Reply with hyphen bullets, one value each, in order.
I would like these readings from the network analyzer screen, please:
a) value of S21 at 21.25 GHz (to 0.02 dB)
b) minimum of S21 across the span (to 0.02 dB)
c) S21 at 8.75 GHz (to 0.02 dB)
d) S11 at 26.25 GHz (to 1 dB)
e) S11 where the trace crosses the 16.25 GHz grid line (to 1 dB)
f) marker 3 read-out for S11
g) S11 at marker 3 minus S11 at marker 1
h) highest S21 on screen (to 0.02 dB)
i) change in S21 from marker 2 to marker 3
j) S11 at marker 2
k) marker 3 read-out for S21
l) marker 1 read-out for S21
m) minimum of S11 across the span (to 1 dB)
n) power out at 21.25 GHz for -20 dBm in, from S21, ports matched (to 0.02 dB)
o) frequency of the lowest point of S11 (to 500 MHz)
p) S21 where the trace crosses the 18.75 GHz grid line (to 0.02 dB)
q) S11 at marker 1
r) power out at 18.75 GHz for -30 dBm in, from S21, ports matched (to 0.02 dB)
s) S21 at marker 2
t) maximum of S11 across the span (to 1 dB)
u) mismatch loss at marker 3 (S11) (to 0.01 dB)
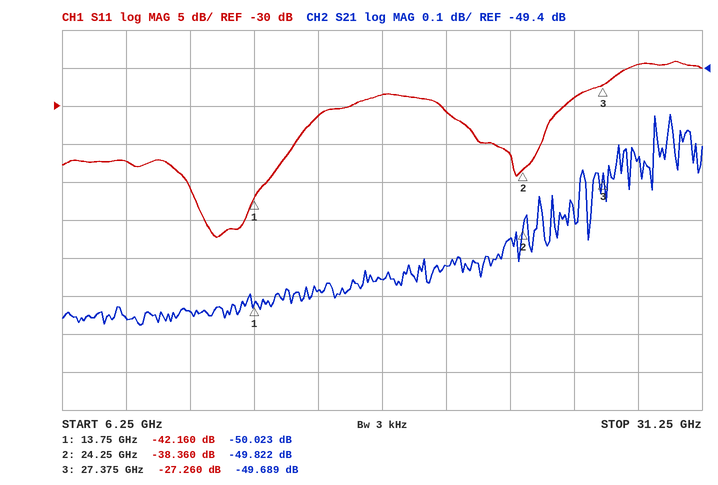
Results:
- -49.92 dB
- -50.08 dB
- -50.06 dB
- -29 dB
- -31 dB
- -27.260 dB
- 14.900 dB
- -49.52 dB
- 0.133 dB
- -38.360 dB
- -49.689 dB
- -50.023 dB
- -47 dB
- -69.92 dBm
- 12.5 GHz
- -49.96 dB
- -42.160 dB
- -79.96 dBm
- -49.822 dB
- -24 dB
- 0.01 dB
